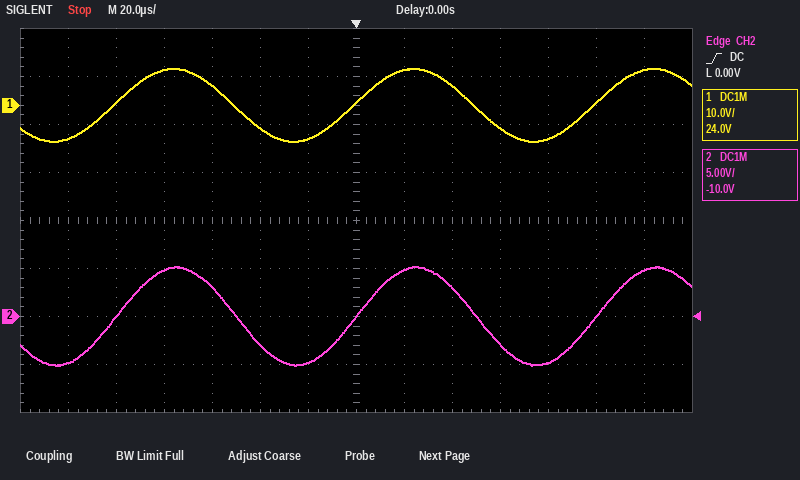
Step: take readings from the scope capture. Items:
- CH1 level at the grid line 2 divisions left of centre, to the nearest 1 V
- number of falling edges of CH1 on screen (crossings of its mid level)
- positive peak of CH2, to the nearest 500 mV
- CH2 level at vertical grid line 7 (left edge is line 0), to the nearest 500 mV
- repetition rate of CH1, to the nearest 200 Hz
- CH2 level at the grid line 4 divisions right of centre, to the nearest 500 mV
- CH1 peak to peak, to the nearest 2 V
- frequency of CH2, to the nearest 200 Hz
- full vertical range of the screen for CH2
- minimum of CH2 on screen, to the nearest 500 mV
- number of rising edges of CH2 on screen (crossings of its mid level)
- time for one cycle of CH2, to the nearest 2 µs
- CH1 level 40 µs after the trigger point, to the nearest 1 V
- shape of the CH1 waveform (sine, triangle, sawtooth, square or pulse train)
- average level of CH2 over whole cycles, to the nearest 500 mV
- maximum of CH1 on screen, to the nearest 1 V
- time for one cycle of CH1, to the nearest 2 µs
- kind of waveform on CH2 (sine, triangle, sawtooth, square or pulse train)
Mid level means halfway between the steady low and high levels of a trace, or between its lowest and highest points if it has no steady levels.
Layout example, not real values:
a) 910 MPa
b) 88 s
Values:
a) -5 V
b) 2
c) 5.0 V
d) 0.0 V
e) 10.0 kHz
f) -5.0 V
g) 16 V
h) 10.0 kHz
i) 40 V
j) -5.0 V
k) 3
l) 100 µs
m) 4 V
n) sine
o) 0.0 V
p) 8 V
q) 100 µs
r) sine
